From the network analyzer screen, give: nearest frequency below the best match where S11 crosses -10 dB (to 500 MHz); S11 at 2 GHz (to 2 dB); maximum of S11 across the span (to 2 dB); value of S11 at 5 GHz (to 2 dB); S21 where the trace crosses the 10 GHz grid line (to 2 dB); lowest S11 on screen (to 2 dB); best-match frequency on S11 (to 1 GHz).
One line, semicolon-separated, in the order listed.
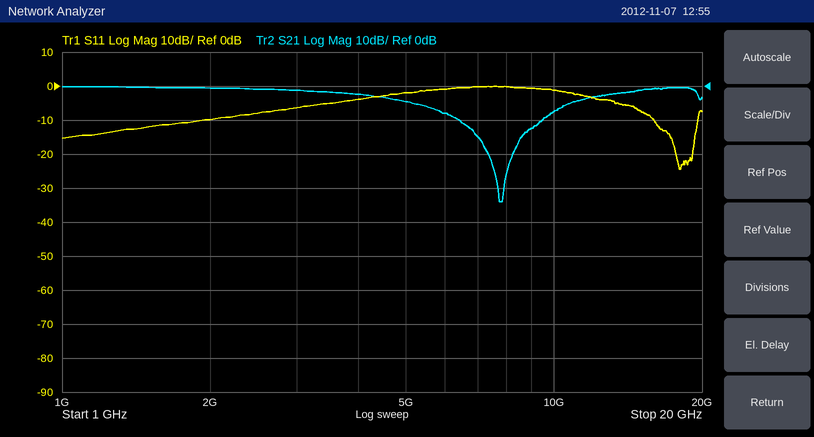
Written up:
16.0 GHz; -10 dB; 0 dB; -2 dB; -8 dB; -24 dB; 18 GHz
